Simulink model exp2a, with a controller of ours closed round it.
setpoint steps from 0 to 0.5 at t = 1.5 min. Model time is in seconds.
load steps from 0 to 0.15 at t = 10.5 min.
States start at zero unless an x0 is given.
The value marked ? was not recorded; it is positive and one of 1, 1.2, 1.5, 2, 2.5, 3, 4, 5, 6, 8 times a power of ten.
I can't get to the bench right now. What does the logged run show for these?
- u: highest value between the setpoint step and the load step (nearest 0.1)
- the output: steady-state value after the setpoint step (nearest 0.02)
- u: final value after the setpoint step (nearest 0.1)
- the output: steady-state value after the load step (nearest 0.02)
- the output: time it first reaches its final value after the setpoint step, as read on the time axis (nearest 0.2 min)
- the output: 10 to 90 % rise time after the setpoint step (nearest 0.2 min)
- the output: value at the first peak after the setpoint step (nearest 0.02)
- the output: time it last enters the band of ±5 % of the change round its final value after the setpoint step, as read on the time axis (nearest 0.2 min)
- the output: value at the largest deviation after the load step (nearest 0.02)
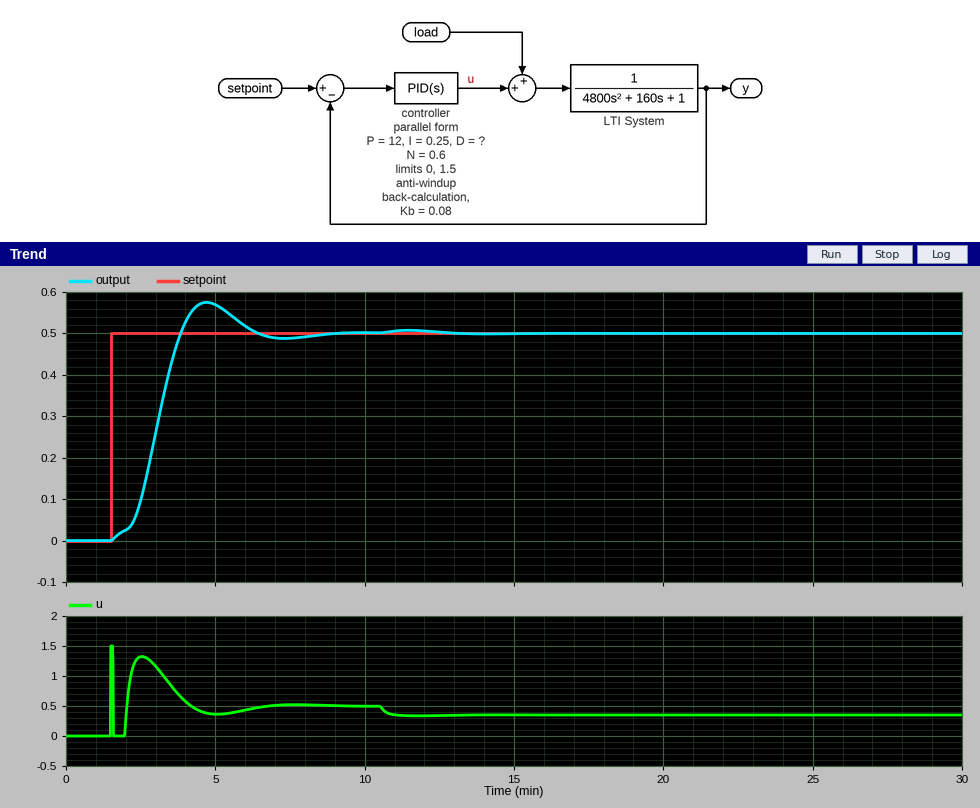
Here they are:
1.5
0.50
0.5
0.50
3.8 min
1.4 min
0.58
5.8 min
0.50
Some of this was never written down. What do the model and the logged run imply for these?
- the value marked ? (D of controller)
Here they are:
400
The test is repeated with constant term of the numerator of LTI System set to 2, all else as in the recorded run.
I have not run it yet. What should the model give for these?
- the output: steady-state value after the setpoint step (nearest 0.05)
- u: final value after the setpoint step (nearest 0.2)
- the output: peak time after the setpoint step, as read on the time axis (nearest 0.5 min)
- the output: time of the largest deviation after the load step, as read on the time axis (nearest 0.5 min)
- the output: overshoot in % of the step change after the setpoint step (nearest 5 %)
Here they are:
0.50
0.2
4.5 min
11.5 min
10 %
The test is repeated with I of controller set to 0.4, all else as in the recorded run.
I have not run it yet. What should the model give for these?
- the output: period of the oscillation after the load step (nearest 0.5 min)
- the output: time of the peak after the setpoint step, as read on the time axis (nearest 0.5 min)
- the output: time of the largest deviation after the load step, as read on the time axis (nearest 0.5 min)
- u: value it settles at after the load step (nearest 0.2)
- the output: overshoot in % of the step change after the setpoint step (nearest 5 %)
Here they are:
4.0 min
4.0 min
11.5 min
0.4
25 %
